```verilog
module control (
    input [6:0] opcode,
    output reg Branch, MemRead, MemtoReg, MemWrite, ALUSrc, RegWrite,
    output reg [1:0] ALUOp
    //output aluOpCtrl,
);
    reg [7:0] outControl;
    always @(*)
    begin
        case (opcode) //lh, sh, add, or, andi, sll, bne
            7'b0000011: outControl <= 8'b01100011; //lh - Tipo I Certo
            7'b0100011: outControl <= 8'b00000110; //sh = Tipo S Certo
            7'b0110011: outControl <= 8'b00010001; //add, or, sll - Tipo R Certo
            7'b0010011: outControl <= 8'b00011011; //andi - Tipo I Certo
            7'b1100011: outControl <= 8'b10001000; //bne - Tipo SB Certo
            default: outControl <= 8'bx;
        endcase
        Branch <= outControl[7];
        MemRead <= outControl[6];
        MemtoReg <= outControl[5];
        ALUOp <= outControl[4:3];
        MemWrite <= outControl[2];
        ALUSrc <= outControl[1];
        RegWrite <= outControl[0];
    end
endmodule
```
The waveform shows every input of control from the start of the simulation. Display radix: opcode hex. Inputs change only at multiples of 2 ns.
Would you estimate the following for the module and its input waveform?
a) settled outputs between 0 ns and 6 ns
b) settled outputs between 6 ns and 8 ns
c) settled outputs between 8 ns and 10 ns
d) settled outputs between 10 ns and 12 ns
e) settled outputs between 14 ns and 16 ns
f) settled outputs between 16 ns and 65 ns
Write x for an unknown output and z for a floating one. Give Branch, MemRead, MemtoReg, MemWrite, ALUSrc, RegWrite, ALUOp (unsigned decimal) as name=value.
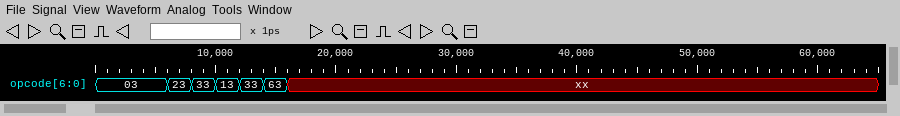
Branch=0, MemRead=1, MemtoReg=1, MemWrite=0, ALUSrc=1, RegWrite=1, ALUOp=0
Branch=0, MemRead=0, MemtoReg=0, MemWrite=1, ALUSrc=1, RegWrite=0, ALUOp=0
Branch=0, MemRead=0, MemtoReg=0, MemWrite=0, ALUSrc=0, RegWrite=1, ALUOp=2
Branch=0, MemRead=0, MemtoReg=0, MemWrite=0, ALUSrc=1, RegWrite=1, ALUOp=3
Branch=1, MemRead=0, MemtoReg=0, MemWrite=0, ALUSrc=0, RegWrite=0, ALUOp=1
Branch=x, MemRead=x, MemtoReg=x, MemWrite=x, ALUSrc=x, RegWrite=x, ALUOp=x
